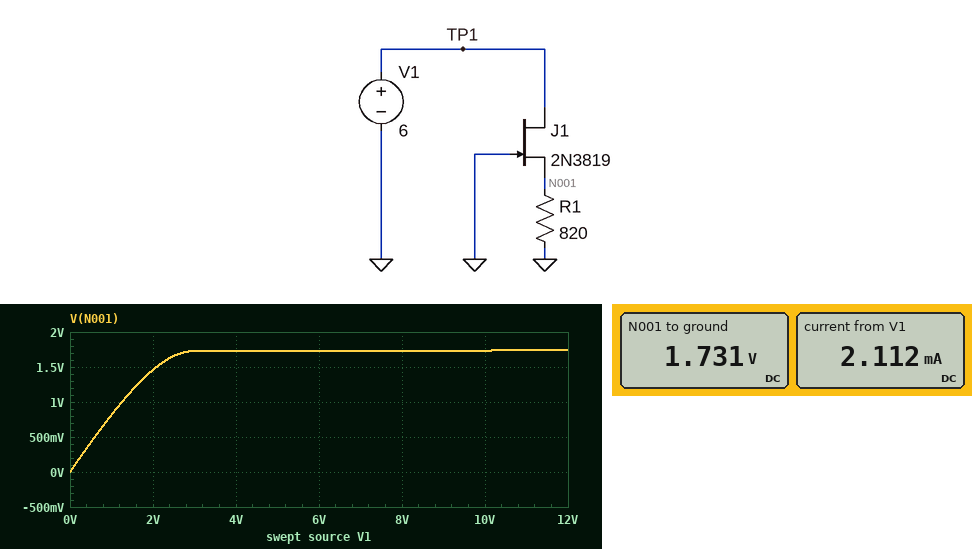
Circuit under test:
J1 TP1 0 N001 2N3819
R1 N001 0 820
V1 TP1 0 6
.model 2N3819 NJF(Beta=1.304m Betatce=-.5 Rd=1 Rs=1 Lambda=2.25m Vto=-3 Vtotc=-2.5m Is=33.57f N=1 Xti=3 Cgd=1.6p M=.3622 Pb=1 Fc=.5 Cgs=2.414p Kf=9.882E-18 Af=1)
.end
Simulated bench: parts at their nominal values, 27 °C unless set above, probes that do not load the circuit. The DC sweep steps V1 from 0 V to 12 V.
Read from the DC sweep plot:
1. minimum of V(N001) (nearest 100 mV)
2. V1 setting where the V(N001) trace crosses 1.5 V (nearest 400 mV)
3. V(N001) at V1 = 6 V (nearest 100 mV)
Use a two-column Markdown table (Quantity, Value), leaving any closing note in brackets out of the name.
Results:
| Quantity | Value |
|---|---|
| minimum of V(N001) | 0 V |
| V1 setting where the V(N001) trace crosses 1.5 V | 2.0 V |
| V(N001) at V1 = 6 V | 1.7 V |
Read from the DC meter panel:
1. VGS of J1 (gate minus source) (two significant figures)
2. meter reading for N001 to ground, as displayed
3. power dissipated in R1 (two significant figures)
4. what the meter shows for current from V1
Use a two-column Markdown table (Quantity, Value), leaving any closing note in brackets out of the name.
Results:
| Quantity | Value |
|---|---|
| VGS of J1 (gate minus source) | -1.7 V |
| meter reading for N001 to ground, as displayed | 1.731 V |
| power dissipated in R1 | 3.7 mW |
| what the meter shows for current from V1 | 2.112 mA |
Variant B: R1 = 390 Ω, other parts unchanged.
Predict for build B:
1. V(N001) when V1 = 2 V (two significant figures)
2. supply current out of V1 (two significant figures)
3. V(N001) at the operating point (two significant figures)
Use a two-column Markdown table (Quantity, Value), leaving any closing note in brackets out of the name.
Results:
| Quantity | Value |
|---|---|
| V(N001) when V1 = 2 V | 1.2 V |
| supply current out of V1 | 3.5 mA |
| V(N001) at the operating point | 1.4 V |
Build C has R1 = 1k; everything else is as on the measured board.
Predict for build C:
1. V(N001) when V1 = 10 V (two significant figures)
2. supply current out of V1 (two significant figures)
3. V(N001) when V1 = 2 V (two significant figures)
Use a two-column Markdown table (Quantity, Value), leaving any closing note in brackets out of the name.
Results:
| Quantity | Value |
|---|---|
| V(N001) when V1 = 10 V | 1.8 V |
| supply current out of V1 | 1.8 mA |
| V(N001) when V1 = 2 V | 1.5 V |
